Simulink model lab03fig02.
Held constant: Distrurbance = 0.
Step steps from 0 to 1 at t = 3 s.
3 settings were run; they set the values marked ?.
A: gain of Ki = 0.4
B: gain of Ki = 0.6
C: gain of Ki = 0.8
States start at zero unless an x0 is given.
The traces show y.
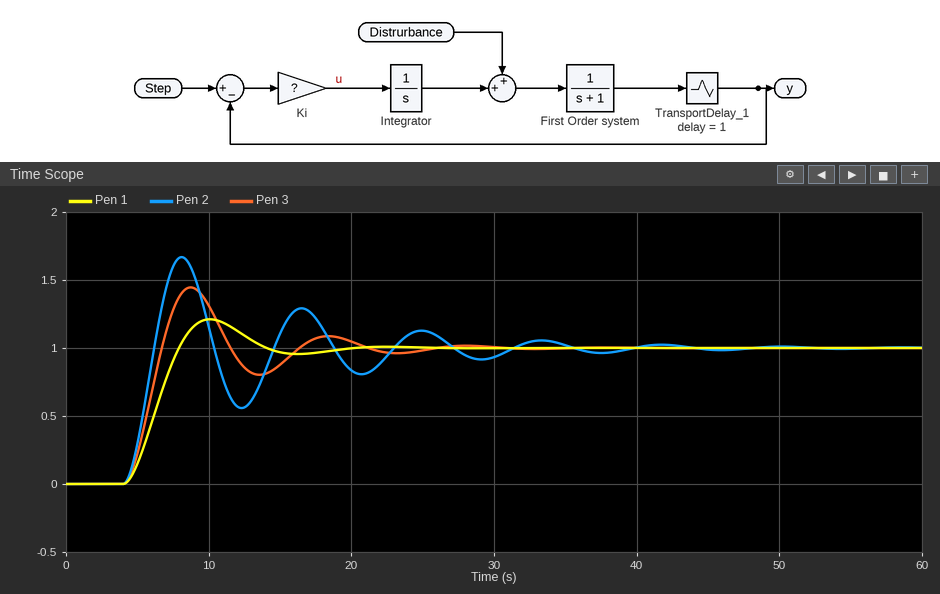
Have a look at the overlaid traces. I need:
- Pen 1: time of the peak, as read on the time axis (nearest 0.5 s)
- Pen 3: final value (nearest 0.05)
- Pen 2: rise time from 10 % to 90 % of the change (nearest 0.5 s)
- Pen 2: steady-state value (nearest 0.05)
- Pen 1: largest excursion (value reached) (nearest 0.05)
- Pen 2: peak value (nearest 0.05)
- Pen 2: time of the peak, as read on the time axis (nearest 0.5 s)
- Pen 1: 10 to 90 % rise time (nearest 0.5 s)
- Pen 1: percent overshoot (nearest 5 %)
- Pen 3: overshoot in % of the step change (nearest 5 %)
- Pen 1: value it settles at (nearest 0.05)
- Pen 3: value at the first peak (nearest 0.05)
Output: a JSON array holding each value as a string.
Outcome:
["10.0 s", "1.00", "1.5 s", "1.00", "1.20", "1.65", "8.0 s", "2.5 s", "20 %", "45 %", "1.00", "1.45"]
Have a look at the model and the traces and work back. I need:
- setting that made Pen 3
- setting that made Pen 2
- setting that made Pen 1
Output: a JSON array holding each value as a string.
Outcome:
["B", "C", "A"]
